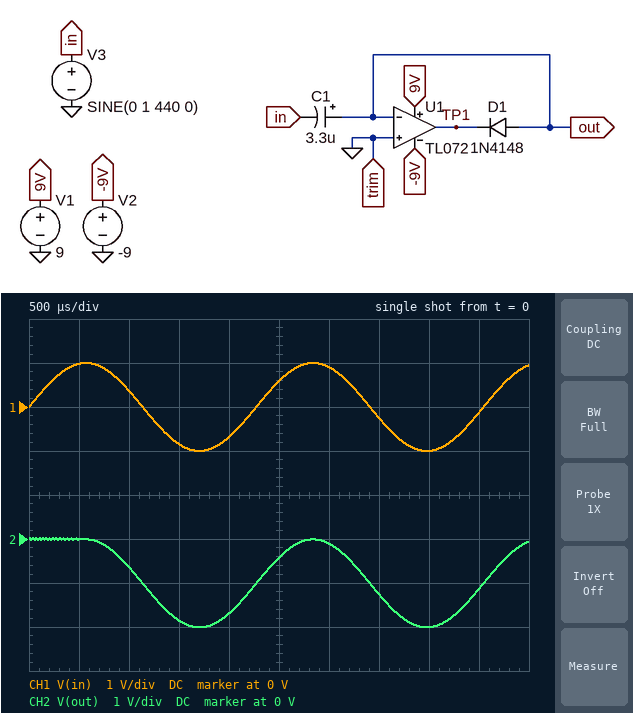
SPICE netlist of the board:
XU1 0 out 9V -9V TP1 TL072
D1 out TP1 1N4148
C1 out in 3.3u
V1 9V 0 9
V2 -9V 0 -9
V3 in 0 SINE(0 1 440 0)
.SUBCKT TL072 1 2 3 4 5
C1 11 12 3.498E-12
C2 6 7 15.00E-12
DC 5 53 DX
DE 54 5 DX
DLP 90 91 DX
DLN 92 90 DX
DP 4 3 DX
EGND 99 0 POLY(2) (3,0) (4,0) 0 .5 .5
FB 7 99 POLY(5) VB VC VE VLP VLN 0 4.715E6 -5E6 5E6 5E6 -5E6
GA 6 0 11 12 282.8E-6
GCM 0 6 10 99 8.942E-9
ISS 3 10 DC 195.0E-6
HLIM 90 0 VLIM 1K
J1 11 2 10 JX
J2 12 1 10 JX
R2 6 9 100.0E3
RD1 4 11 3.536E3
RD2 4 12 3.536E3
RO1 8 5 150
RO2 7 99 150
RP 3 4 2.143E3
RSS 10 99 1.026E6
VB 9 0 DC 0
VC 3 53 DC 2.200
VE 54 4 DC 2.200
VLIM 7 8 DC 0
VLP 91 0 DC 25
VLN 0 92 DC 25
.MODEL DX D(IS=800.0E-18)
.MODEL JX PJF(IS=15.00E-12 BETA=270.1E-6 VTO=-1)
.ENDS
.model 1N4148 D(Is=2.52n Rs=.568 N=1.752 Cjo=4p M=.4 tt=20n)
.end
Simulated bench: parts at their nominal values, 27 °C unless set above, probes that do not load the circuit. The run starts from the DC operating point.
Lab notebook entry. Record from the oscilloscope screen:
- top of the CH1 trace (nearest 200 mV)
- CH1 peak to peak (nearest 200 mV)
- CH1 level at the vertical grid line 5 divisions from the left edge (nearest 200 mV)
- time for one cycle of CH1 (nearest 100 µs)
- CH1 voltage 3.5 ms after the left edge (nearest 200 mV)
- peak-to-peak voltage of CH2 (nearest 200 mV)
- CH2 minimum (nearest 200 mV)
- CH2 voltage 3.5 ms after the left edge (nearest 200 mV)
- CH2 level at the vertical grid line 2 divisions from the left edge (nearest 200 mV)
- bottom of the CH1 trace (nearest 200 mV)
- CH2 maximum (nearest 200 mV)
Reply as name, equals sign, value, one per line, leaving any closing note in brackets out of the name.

top of the CH1 trace = 1.0 V
CH1 peak to peak = 2.0 V
CH1 level at the vertical grid line 5 divisions from the left edge = 600 mV
time for one cycle of CH1 = 2.3 ms
CH1 voltage 3.5 ms after the left edge = -200 mV
peak-to-peak voltage of CH2 = 2.0 V
CH2 minimum = -2.0 V
CH2 voltage 3.5 ms after the left edge = -1.2 V
CH2 level at the vertical grid line 2 divisions from the left edge = -600 mV
bottom of the CH1 trace = -1.0 V
CH2 maximum = 0 V
